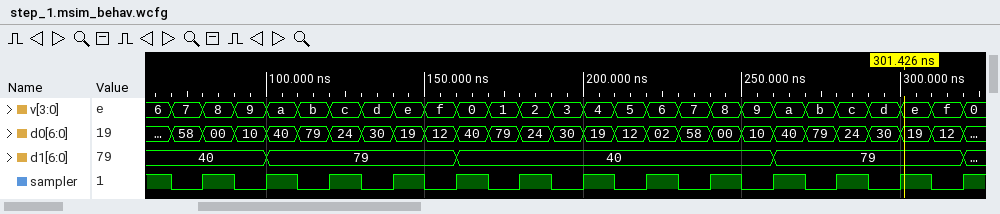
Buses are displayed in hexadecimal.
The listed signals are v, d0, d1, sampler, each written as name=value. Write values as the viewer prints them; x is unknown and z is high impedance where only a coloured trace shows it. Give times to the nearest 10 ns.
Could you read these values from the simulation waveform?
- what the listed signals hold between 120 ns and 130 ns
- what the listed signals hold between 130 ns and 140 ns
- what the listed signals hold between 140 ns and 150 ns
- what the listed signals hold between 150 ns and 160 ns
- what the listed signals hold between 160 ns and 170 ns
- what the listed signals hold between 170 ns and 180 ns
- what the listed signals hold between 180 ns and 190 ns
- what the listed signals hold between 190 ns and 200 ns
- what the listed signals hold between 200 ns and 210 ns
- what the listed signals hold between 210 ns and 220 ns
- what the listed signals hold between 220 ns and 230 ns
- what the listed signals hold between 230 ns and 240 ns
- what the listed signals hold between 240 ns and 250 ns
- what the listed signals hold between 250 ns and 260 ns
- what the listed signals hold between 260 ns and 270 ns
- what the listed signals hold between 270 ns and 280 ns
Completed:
v=c, d0=24, d1=79, sampler=1
v=d, d0=30, d1=79, sampler=0
v=e, d0=19, d1=79, sampler=1
v=f, d0=12, d1=79, sampler=0
v=0, d0=40, d1=40, sampler=1
v=1, d0=79, d1=40, sampler=0
v=2, d0=24, d1=40, sampler=1
v=3, d0=30, d1=40, sampler=0
v=4, d0=19, d1=40, sampler=1
v=5, d0=12, d1=40, sampler=0
v=6, d0=02, d1=40, sampler=1
v=7, d0=58, d1=40, sampler=0
v=8, d0=00, d1=40, sampler=1
v=9, d0=10, d1=40, sampler=0
v=a, d0=40, d1=79, sampler=1
v=b, d0=79, d1=79, sampler=0
